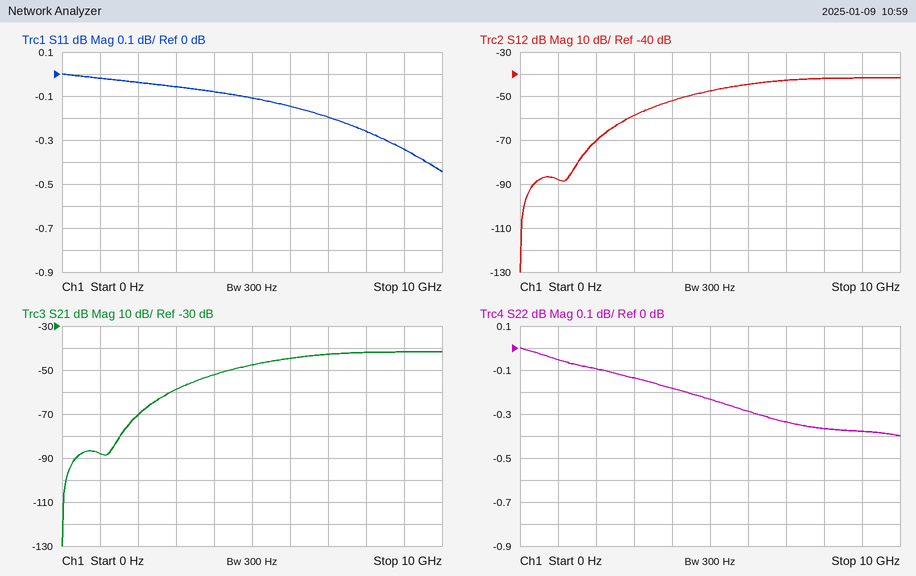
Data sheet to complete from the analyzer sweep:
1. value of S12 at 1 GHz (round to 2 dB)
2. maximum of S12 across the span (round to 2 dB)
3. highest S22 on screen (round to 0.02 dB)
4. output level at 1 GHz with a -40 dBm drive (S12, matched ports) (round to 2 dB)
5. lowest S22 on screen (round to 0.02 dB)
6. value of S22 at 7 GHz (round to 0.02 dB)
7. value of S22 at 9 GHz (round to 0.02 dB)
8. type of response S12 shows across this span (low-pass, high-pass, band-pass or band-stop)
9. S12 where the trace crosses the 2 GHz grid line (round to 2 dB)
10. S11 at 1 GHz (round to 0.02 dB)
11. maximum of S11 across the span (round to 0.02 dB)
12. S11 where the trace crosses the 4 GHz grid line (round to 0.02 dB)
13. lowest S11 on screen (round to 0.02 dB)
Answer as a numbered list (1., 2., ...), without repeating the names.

1. -88 dB
2. -42 dB
3. 0.00 dB
4. -128 dBm
5. -0.40 dB
6. -0.34 dB
7. -0.38 dB
8. high-pass
9. -70 dB
10. -0.02 dB
11. 0.00 dB
12. -0.08 dB
13. -0.44 dB
